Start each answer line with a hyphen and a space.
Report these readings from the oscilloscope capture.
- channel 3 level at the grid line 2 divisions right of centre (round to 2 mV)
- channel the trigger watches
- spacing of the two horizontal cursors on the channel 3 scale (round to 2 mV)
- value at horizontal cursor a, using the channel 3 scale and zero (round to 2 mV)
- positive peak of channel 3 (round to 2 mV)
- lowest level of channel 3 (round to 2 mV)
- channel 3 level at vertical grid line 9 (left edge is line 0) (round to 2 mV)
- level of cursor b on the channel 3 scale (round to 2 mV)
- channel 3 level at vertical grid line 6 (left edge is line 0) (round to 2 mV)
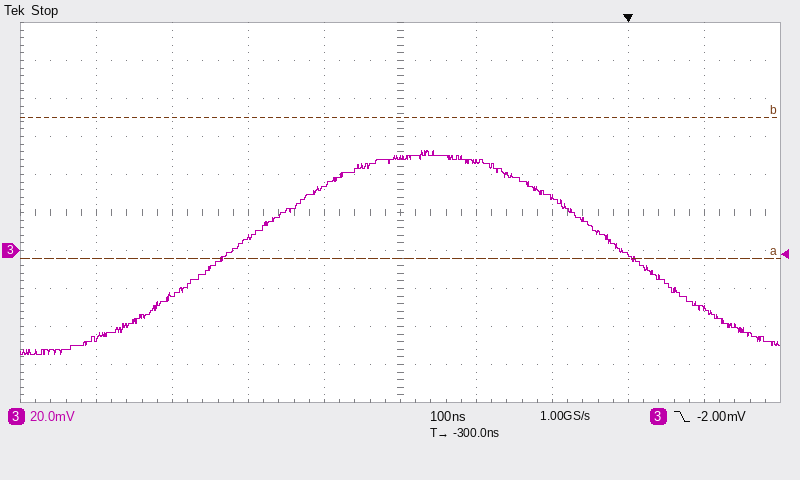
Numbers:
- 28 mV
- channel 3
- 74 mV
- -4 mV
- 52 mV
- -54 mV
- -30 mV
- 70 mV
- 46 mV
